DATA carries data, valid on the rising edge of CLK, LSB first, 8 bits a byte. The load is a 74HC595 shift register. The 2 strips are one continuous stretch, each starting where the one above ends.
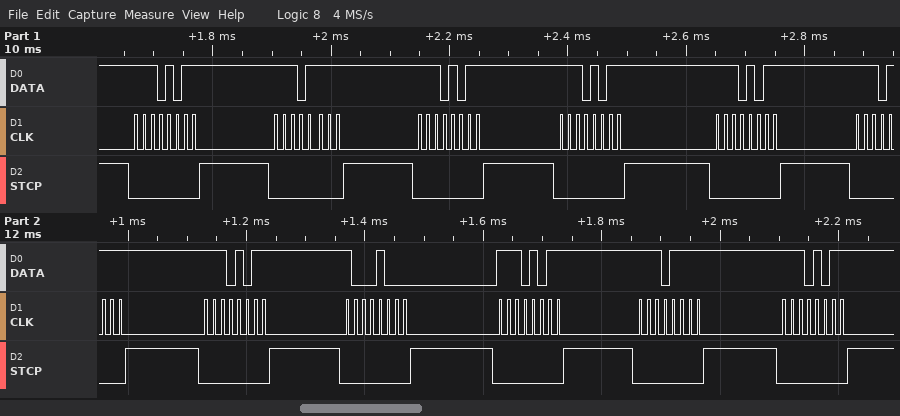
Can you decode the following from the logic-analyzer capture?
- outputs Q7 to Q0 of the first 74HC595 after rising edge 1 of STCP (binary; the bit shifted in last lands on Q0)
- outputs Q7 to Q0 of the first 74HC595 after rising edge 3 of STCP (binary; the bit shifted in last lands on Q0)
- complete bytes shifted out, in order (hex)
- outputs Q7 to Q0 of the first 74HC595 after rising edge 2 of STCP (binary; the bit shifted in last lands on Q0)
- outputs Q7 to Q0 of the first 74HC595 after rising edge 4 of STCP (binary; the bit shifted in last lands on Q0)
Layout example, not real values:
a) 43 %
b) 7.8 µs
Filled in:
a) 11101011
b) 11101011
c) D7 F7 D7 D7 D7 F7 D7 11 D7 F7 D7
d) 11101111
e) 11101011
